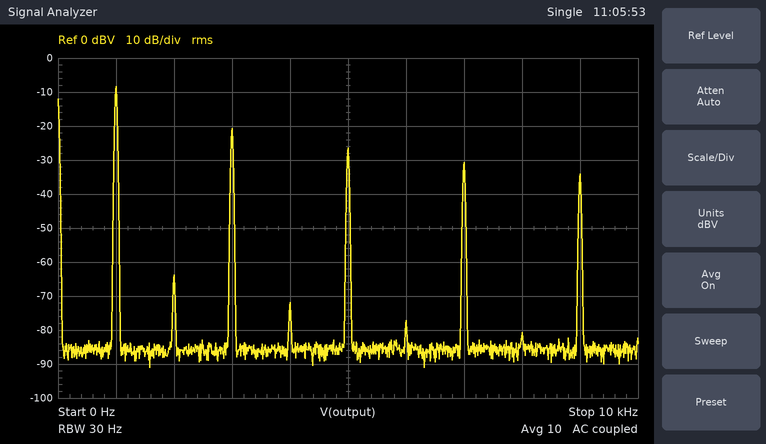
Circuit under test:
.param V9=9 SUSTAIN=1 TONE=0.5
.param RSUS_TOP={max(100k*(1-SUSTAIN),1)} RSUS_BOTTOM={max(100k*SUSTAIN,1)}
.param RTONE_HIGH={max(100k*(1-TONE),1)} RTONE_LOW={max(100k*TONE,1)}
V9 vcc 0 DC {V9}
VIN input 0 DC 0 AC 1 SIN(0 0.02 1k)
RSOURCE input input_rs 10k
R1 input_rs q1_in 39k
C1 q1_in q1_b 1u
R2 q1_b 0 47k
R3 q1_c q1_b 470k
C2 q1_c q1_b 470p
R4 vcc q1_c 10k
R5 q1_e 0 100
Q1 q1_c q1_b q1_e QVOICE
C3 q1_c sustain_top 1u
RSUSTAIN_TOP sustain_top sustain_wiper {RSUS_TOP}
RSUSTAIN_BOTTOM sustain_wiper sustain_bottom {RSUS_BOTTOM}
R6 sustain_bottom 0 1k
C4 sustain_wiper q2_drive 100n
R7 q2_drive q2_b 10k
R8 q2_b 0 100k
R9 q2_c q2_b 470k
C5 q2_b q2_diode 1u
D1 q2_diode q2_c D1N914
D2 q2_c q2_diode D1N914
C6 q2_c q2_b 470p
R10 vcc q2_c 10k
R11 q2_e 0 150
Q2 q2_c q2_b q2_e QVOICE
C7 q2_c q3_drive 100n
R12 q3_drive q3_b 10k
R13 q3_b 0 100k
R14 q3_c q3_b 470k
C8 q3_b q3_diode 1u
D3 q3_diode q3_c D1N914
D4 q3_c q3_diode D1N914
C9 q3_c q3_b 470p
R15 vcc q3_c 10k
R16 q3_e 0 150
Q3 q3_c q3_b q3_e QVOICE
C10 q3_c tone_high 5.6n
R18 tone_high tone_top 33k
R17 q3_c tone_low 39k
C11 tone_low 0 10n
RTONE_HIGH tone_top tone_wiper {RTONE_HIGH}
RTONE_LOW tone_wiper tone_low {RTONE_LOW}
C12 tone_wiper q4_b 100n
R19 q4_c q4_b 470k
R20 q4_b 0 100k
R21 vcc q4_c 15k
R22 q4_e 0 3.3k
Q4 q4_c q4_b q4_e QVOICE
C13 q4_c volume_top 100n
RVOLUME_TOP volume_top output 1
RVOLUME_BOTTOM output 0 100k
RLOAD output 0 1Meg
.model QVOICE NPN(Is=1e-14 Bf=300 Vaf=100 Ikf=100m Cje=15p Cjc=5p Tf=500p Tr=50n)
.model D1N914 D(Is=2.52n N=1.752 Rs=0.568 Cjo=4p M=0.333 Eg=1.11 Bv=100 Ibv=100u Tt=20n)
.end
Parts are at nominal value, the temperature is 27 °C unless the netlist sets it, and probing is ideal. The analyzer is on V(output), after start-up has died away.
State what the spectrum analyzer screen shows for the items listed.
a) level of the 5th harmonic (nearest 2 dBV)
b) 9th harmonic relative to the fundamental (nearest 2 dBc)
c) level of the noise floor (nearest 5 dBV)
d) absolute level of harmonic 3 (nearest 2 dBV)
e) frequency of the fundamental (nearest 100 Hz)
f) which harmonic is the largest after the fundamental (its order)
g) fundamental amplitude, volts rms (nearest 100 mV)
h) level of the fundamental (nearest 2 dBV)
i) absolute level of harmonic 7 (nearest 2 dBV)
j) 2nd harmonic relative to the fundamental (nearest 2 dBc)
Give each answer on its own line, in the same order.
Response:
-26 dBV
-26 dBc
-85 dBV
-20 dBV
1.0 kHz
3
400 mV
-8 dBV
-30 dBV
-56 dBc
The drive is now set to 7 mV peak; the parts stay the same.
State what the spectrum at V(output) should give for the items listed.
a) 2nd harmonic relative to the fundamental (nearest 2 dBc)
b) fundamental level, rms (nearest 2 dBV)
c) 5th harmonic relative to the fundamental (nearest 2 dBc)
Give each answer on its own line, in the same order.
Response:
-52 dBc
-8 dBV
-20 dBc
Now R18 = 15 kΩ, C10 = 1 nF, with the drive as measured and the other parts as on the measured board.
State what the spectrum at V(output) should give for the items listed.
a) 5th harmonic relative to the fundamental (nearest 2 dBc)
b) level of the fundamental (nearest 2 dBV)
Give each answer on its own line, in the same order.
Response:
-12 dBc
-14 dBV
